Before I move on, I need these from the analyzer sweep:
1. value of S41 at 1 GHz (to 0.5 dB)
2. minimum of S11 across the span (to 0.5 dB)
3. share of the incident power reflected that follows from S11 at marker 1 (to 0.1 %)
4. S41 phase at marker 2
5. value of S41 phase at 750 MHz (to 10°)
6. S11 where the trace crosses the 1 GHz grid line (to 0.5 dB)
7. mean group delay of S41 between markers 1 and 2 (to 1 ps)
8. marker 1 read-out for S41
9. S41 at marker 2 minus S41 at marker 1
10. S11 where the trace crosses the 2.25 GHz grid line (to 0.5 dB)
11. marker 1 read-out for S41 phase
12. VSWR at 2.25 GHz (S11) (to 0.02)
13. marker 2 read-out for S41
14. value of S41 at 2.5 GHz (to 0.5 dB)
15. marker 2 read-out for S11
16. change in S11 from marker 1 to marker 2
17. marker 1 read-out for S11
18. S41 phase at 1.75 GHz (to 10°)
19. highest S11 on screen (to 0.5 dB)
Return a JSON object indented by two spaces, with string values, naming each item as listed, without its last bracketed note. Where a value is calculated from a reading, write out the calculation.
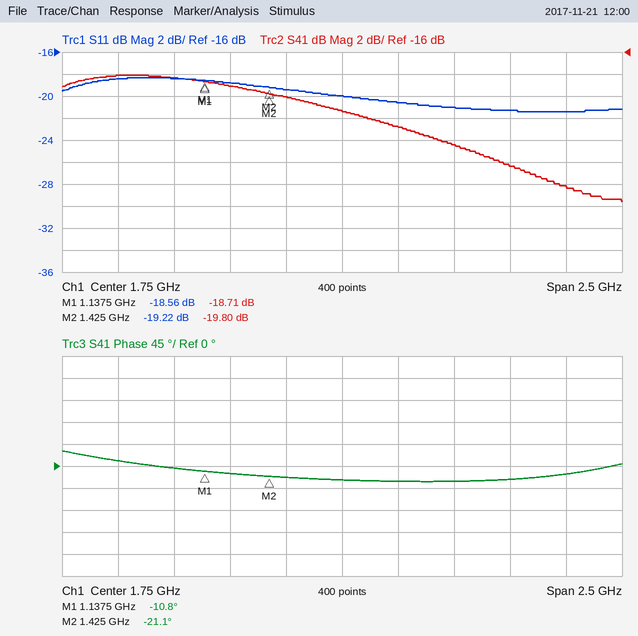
{
  "value of S41 at 1 GHz": "-18.5 dB",
  "minimum of S11 across the span": "-21.5 dB",
  "share of the incident power reflected that follows from S11 at marker 1": "10^(-18.56/10) ≈ 1.4 %",
  "S41 phase at marker 2": "-21.1°",
  "value of S41 phase at 750 MHz": "10°",
  "S11 where the trace crosses the 1 GHz grid line": "-18.5 dB",
  "mean group delay of S41 between markers 1 and 2": "−(-21.1° − (-10.8°))/(360° × 287.5 MHz) ≈ 100 ps",
  "marker 1 read-out for S41": "-18.71 dB",
  "S41 at marker 2 minus S41 at marker 1": "-19.8 − (-18.71) = -1.09 dB",
  "S11 where the trace crosses the 2.25 GHz grid line": "-21.0 dB",
  "marker 1 read-out for S41 phase": "-10.8°",
  "VSWR at 2.25 GHz (S11)": "|Γ| = 10^(-21/20) = 0.0891; VSWR = (1 + 0.0891)/(1 − 0.0891) ≈ 1.20",
  "marker 2 read-out for S41": "-19.80 dB",
  "value of S41 at 2.5 GHz": "-26.5 dB",
  "marker 2 read-out for S11": "-19.22 dB",
  "change in S11 from marker 1 to marker 2": "-19.22 − (-18.56) = -0.66 dB",
  "marker 1 read-out for S11": "-18.56 dB",
  "S41 phase at 1.75 GHz": "-30°",
  "highest S11 on screen": "-18.5 dB"
}
